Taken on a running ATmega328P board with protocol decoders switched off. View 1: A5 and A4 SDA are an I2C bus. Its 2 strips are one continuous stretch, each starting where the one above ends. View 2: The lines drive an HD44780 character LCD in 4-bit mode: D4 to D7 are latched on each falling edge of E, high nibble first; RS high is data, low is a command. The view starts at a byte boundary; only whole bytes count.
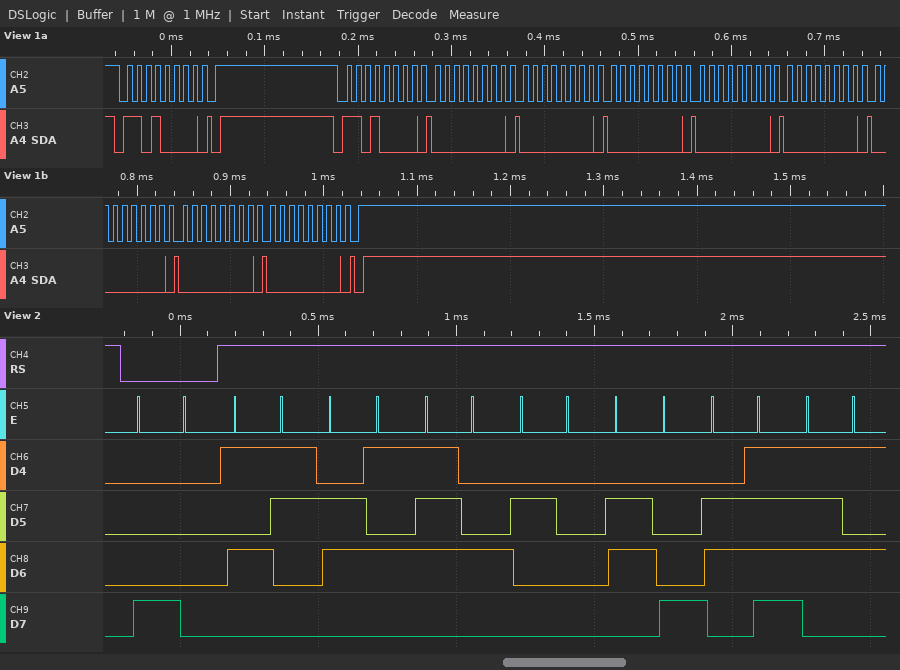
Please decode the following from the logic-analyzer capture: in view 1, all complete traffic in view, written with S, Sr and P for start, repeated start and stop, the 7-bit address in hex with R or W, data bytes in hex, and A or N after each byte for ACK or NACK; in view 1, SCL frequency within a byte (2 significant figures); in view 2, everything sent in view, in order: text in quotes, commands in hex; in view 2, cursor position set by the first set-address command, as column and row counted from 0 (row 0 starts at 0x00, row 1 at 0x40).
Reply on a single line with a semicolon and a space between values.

S 68W A P S 68W A 00 A 00 A 00 A 00 A 00 A 00 A 00 A 00 A P; 100 kHz; 0x80 "Set hou"; column 0, row 0
